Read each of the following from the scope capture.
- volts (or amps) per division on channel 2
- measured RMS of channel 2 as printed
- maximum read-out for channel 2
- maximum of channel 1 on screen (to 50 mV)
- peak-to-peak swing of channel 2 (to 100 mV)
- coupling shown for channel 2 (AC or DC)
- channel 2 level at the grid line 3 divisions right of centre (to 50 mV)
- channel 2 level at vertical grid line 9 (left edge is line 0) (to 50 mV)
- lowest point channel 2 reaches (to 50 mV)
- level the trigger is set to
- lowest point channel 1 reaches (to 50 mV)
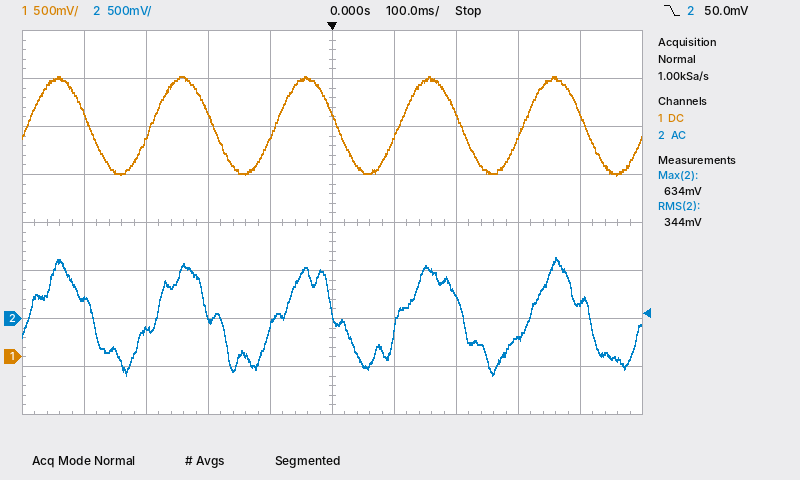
500 mV
344 mV
634 mV
2.90 V
1.20 V
AC
-200 mV
150 mV
-600 mV
50.0 mV
1.90 V
